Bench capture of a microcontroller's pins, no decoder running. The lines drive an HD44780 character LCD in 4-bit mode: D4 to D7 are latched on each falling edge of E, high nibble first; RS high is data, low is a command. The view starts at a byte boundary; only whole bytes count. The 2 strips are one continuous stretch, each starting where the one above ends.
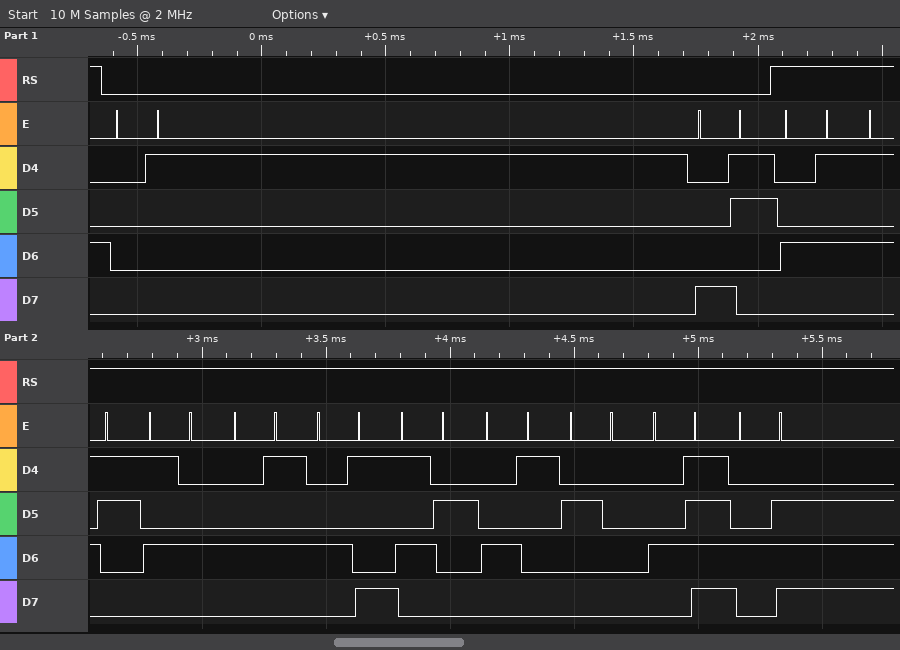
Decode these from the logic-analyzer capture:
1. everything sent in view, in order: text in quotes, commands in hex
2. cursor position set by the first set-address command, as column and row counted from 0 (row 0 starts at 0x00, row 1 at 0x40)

0x01 0x83 "ESTEIRA ON"
column 3, row 0
